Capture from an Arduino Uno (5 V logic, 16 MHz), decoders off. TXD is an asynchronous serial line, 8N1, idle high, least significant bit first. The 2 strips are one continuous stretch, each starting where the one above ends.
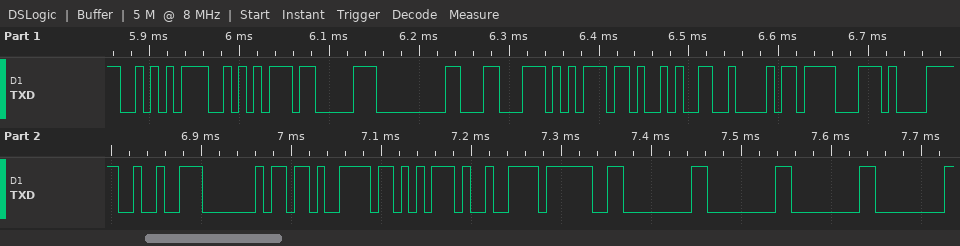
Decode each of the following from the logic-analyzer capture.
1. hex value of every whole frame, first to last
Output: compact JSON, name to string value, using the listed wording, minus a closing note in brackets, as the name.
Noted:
{"hex value of every whole frame, first to last": "AA AA 83 00 8C 75 29 42 8F E1 92 40 CB AB C9 3F 00 00 00 00"}
